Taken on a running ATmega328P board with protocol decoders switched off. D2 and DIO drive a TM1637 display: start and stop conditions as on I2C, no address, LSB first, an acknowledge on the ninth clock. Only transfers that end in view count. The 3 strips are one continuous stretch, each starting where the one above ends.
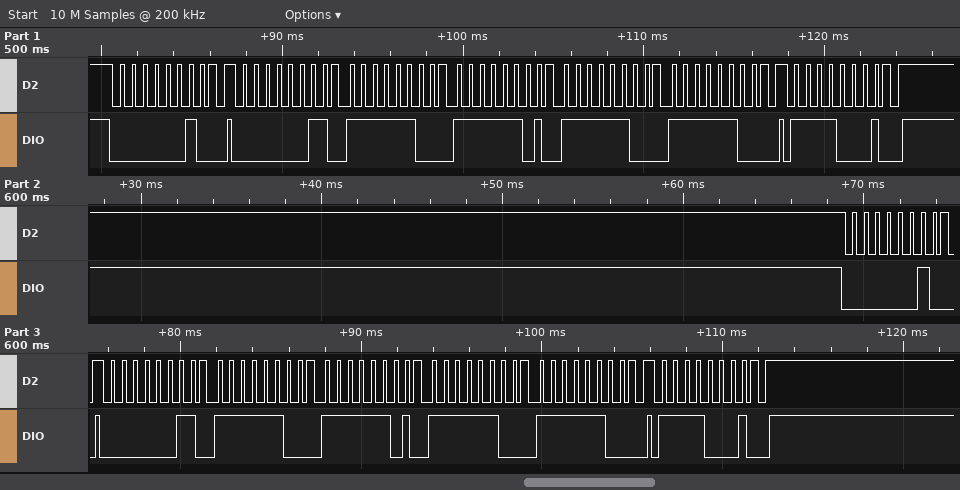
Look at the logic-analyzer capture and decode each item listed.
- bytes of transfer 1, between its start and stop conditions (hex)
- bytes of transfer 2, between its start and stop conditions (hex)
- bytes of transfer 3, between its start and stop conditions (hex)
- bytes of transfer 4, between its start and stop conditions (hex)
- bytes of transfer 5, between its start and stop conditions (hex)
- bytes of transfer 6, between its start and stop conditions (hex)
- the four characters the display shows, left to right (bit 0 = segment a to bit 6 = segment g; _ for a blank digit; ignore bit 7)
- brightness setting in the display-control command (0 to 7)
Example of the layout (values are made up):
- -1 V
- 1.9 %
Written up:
- 40
- C0 3F BF 3F 3F
- 8F
- 40
- C0 3F BF 3F 3F
- 8F
- 0000
- 7
